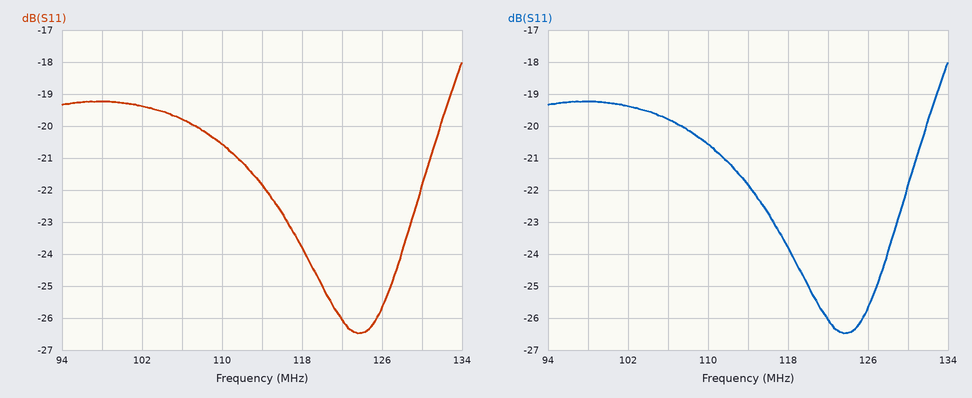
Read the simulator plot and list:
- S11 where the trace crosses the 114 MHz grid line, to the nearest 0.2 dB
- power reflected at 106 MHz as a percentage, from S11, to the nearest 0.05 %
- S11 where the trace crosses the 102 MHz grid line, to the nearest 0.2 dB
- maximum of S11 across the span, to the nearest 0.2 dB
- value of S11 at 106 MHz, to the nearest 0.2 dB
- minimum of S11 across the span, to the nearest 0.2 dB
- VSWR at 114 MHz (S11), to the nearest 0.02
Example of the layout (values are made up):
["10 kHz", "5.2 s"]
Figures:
["-21.8 dB", "1.05 %", "-19.4 dB", "-18.0 dB", "-19.8 dB", "-26.4 dB", "1.18"]
